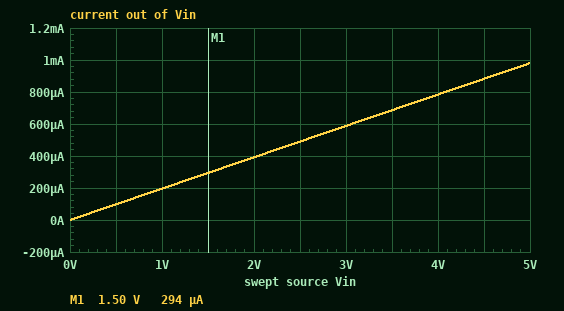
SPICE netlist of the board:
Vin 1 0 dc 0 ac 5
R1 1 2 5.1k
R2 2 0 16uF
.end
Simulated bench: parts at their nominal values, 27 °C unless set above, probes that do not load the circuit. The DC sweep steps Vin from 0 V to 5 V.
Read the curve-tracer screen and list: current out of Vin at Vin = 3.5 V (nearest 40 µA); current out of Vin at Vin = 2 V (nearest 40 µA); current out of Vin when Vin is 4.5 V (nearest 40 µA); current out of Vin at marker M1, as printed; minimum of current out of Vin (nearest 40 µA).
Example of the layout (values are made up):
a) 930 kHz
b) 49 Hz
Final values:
a) 680 µA
b) 400 µA
c) 880 µA
d) 294 µA
e) 0 A
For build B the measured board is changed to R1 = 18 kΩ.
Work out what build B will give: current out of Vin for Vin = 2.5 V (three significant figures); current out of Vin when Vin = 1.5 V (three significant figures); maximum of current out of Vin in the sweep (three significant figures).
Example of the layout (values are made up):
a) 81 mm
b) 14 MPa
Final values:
a) 139 µA
b) 83.3 µA
c) 278 µA
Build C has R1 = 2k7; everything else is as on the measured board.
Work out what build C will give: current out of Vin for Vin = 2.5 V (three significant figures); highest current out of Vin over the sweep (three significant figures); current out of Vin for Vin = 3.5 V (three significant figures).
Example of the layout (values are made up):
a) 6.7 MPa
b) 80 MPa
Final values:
a) 926 µA
b) 1.85 mA
c) 1.30 mA
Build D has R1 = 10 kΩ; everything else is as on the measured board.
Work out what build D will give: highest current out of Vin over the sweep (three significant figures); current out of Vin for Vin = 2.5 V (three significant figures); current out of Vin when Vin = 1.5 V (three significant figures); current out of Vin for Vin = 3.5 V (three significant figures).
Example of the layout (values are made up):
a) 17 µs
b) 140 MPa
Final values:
a) 500 µA
b) 250 µA
c) 150 µA
d) 350 µA
